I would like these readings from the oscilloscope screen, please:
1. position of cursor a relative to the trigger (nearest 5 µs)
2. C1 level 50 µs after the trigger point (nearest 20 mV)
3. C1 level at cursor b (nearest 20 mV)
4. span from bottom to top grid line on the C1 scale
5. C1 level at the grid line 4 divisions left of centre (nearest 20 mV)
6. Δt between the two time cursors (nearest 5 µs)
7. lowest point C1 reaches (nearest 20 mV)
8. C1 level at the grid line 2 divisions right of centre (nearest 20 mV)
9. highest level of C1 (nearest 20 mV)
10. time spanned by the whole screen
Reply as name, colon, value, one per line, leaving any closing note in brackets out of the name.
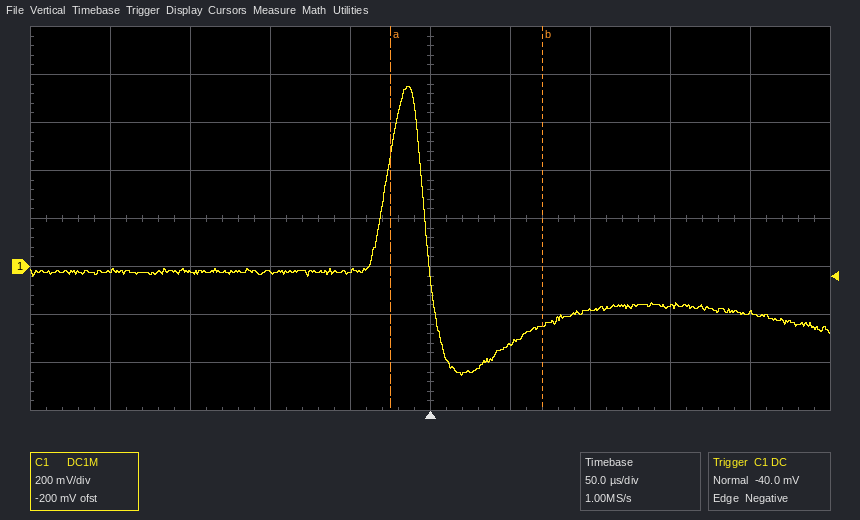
position of cursor a relative to the trigger: -25 µs
C1 level 50 µs after the trigger point: -320 mV
C1 level at cursor b: -240 mV
span from bottom to top grid line on the C1 scale: 1.6 V
C1 level at the grid line 4 divisions left of centre: -20 mV
Δt between the two time cursors: 95 µs
lowest point C1 reaches: -460 mV
C1 level at the grid line 2 divisions right of centre: -180 mV
highest level of C1: 760 mV
time spanned by the whole screen: 500 µs
